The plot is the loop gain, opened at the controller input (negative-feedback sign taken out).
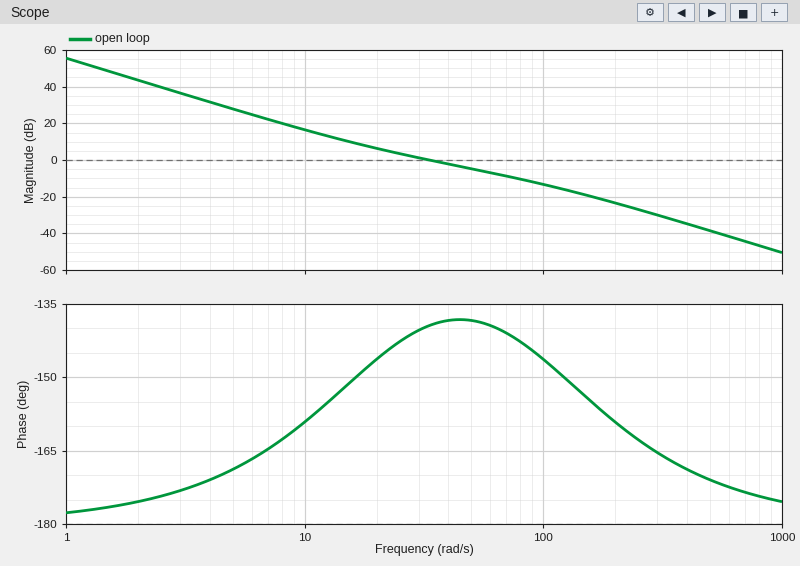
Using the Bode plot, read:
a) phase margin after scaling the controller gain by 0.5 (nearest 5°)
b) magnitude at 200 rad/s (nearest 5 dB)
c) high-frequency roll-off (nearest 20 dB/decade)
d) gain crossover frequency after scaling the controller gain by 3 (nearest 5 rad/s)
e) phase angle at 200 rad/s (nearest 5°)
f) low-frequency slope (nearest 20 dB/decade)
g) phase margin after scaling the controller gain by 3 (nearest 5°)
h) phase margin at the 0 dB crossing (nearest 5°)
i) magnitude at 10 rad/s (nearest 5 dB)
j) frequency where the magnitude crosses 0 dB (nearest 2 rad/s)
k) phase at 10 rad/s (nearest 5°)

35°
-25 dB
-40 dB/decade
75 rad/s
-160°
-40 dB/decade
40°
40°
15 dB
34 rad/s
-160°
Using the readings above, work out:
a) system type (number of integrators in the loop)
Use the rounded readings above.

2
